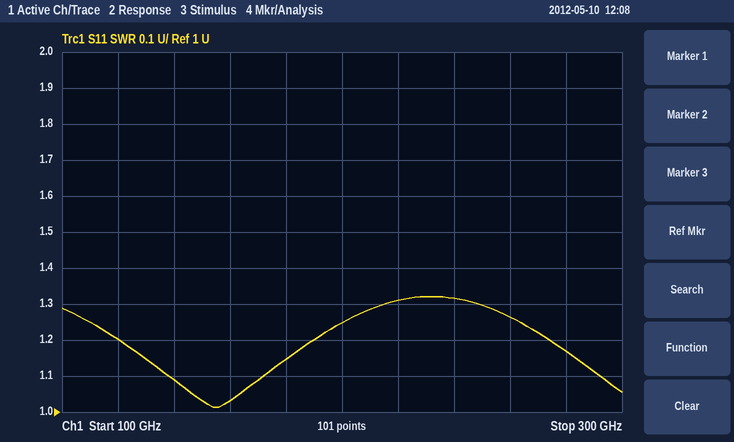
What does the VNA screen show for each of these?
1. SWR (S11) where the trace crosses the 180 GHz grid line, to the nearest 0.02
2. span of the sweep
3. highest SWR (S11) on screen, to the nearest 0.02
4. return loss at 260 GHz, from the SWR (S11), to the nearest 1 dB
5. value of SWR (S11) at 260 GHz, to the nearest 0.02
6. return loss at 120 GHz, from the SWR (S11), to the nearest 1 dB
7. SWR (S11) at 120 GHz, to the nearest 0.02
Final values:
1.14
200 GHz
1.32
19 dB
1.26
21 dB
1.20
